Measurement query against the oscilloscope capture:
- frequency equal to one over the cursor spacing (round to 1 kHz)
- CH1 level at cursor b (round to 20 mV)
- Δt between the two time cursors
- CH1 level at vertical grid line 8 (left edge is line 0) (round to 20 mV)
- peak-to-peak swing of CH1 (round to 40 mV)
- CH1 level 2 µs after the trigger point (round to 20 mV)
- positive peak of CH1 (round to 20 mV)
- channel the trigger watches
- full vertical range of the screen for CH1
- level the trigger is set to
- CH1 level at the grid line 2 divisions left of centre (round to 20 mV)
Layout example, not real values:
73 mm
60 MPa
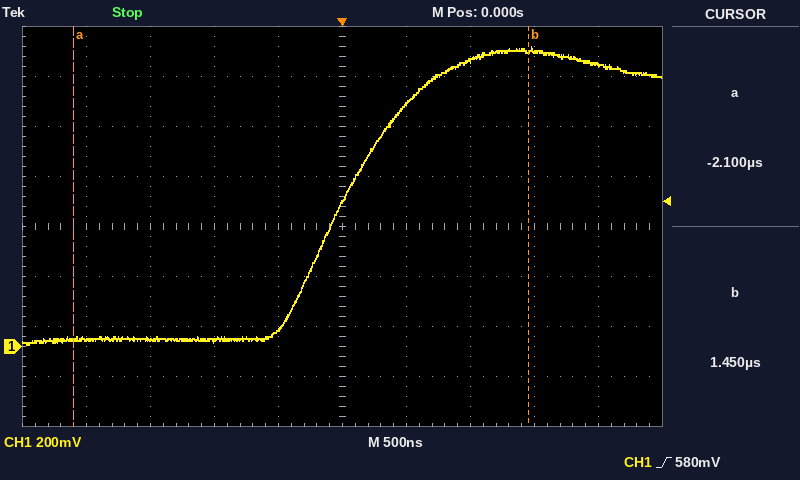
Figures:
282 kHz
1.18 V
3.55 µs
1.18 V
1.20 V
1.12 V
1.20 V
CH1
1.6 V
580 mV
20 mV
